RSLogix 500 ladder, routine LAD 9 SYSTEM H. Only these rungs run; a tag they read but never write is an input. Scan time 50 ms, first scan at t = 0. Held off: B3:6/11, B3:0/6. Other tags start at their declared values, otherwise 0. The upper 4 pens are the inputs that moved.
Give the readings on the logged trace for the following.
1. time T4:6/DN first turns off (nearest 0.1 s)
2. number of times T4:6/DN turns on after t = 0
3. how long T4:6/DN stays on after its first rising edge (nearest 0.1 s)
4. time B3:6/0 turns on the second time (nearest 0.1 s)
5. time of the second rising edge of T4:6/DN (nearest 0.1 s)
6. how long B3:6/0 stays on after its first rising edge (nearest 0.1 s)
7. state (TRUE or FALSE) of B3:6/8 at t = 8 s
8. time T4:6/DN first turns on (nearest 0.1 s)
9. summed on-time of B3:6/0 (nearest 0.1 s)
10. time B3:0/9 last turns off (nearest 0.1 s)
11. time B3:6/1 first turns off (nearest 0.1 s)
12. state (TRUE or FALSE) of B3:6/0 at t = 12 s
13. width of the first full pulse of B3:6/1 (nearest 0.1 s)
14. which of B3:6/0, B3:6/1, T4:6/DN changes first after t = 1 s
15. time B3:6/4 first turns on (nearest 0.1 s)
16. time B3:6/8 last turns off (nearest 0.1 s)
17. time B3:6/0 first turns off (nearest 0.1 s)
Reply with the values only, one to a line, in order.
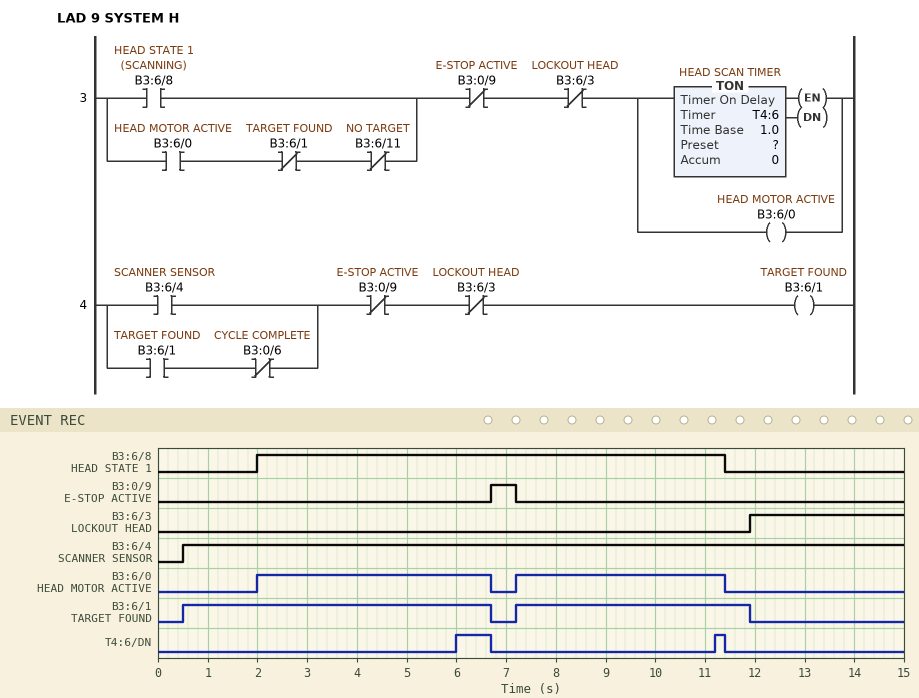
6.7 s
2
0.7 s
7.2 s
11.2 s
4.7 s
TRUE
6.0 s
8.9 s
7.2 s
6.7 s
FALSE
6.2 s
B3:6/0
0.5 s
11.4 s
6.7 s
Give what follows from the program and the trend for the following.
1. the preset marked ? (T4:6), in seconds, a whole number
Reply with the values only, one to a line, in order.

4 s
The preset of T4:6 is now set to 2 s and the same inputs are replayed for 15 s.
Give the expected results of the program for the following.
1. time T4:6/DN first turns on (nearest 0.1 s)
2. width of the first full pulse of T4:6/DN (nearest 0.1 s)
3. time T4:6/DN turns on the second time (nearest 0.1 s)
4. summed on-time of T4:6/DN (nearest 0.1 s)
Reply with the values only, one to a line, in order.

4.0 s
2.7 s
9.2 s
4.9 s
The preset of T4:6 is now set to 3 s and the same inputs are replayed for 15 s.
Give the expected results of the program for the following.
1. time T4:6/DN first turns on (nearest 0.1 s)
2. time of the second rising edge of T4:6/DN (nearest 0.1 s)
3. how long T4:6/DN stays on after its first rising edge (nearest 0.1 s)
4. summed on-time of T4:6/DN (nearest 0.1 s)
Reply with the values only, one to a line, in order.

5.0 s
10.2 s
1.7 s
2.9 s
